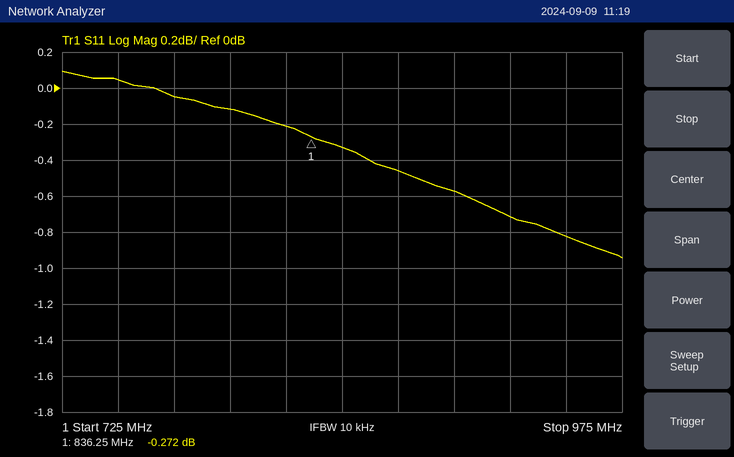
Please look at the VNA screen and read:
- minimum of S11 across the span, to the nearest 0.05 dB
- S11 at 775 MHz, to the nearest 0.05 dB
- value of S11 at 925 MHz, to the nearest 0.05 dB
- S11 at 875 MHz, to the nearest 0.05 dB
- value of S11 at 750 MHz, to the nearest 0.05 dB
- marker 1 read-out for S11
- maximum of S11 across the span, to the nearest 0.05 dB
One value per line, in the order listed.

-0.95 dB
-0.05 dB
-0.70 dB
-0.45 dB
0.05 dB
-0.272 dB
0.10 dB
